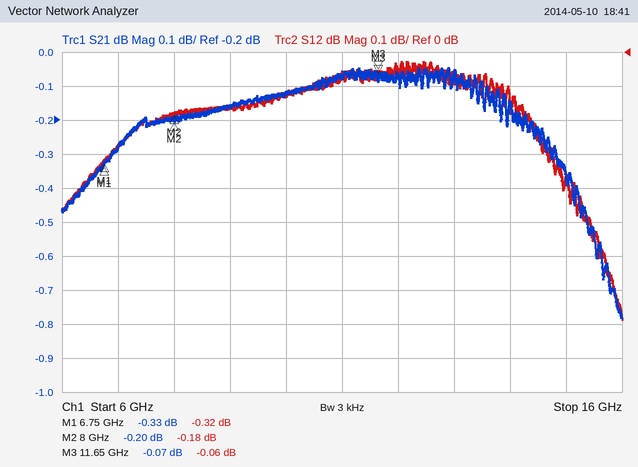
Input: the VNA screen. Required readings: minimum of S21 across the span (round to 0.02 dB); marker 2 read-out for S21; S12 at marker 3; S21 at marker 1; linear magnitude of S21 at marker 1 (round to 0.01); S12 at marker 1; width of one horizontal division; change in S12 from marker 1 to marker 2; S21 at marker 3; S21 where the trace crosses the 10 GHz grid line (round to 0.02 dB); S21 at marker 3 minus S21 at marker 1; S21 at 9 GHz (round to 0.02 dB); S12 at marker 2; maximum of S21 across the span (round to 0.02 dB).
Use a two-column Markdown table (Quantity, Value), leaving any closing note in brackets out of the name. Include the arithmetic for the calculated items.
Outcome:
| Quantity | Value |
|---|---|
| minimum of S21 across the span | -0.78 dB |
| marker 2 read-out for S21 | -0.20 dB |
| S12 at marker 3 | -0.06 dB |
| S21 at marker 1 | -0.33 dB |
| linear magnitude of S21 at marker 1 | 10^(-0.33/20) ≈ 0.96 |
| S12 at marker 1 | -0.32 dB |
| width of one horizontal division | 1 GHz |
| change in S12 from marker 1 to marker 2 | -0.18 − (-0.32) = 0.14 dB |
| S21 at marker 3 | -0.07 dB |
| S21 where the trace crosses the 10 GHz grid line | -0.12 dB |
| S21 at marker 3 minus S21 at marker 1 | -0.07 − (-0.33) = 0.26 dB |
| S21 at 9 GHz | -0.16 dB |
| S12 at marker 2 | -0.18 dB |
| maximum of S21 across the span | -0.04 dB |
